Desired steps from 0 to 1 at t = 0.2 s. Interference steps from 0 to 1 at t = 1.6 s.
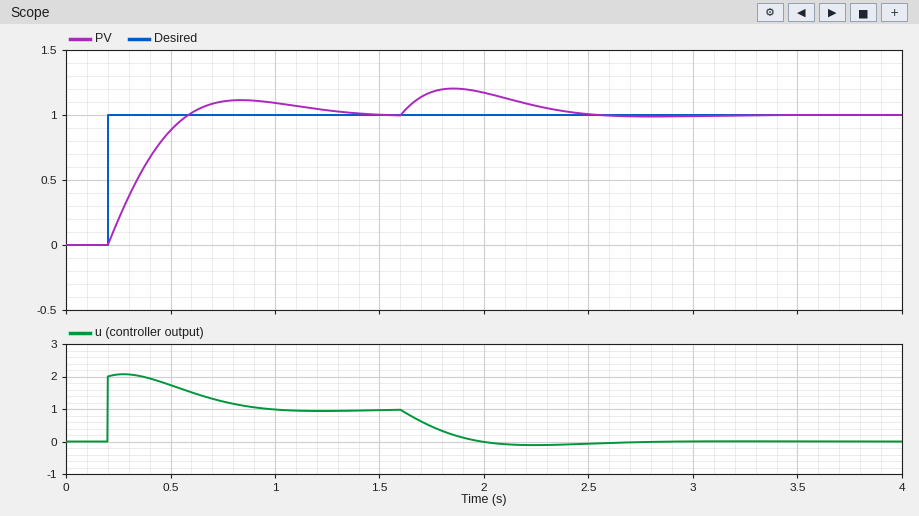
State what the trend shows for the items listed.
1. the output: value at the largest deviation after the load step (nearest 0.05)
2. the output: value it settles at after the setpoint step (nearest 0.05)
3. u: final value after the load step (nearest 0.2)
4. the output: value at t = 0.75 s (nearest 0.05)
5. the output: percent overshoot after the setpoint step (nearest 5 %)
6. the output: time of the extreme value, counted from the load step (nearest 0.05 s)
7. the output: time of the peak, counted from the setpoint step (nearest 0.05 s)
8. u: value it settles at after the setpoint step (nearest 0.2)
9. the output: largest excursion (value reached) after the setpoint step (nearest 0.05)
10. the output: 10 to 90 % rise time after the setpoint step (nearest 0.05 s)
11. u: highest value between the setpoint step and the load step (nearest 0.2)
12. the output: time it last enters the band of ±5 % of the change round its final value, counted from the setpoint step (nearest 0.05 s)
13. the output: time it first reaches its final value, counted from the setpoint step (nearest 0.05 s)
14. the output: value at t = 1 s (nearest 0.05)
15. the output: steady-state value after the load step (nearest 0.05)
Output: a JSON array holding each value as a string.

["1.20", "1.00", "0.0", "1.10", "10 %", "0.25 s", "0.65 s", "1.0", "1.10", "0.30 s", "2.0", "1.00 s", "0.40 s", "1.10", "1.00"]
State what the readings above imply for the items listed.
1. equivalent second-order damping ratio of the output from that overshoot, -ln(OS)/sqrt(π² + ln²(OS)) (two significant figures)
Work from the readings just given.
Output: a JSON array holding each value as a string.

["0.59"]
